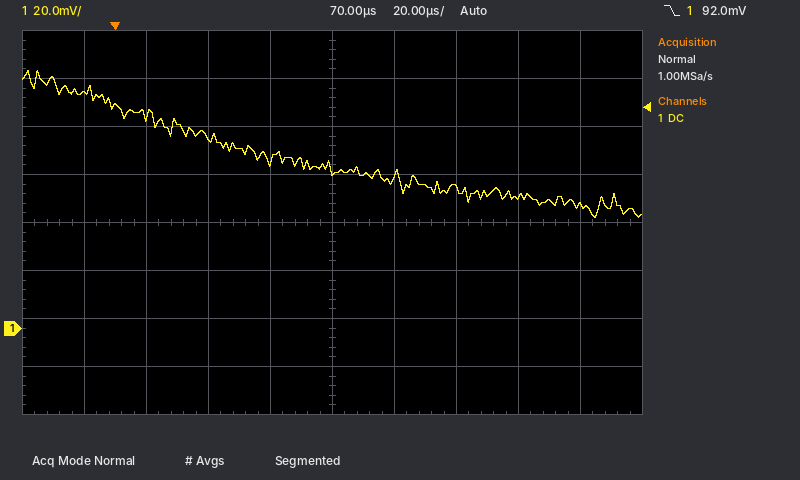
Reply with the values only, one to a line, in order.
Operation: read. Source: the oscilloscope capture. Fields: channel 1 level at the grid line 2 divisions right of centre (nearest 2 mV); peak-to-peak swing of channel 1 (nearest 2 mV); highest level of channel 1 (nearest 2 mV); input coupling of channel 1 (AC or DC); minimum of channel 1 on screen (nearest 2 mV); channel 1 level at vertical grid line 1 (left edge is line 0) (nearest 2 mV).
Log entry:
58 mV
62 mV
108 mV
DC
46 mV
98 mV
